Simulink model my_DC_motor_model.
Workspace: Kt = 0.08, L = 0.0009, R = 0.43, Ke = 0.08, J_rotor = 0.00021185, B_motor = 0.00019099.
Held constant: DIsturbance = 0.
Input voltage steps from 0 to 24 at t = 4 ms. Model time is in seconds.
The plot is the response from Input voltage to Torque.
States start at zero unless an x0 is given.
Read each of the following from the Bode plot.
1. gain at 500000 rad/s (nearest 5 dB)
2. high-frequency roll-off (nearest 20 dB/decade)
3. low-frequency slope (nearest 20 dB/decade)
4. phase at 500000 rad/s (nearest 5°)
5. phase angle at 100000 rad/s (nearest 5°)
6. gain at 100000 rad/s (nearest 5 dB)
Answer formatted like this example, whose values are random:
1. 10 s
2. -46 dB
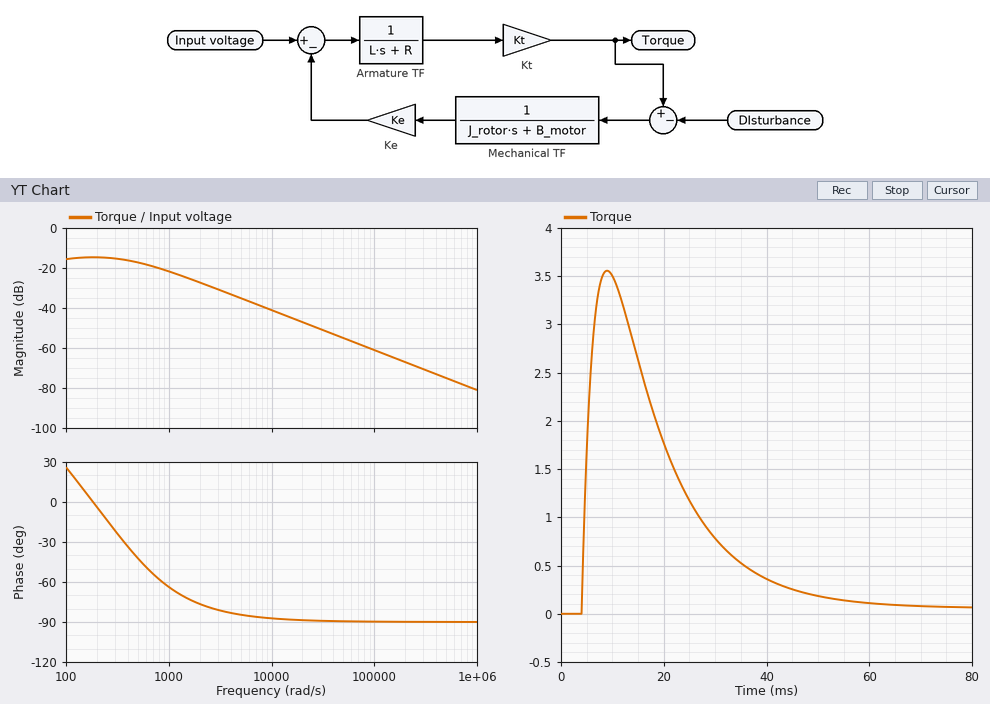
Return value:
1. -75 dB
2. -20 dB/decade
3. 0 dB/decade
4. -90°
5. -90°
6. -60 dB
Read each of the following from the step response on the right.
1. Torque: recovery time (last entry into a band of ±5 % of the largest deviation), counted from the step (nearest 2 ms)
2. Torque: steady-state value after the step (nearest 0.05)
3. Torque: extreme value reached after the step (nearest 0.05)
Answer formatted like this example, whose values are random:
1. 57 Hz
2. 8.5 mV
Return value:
1. 42 ms
2. 0.05
3. 3.55
